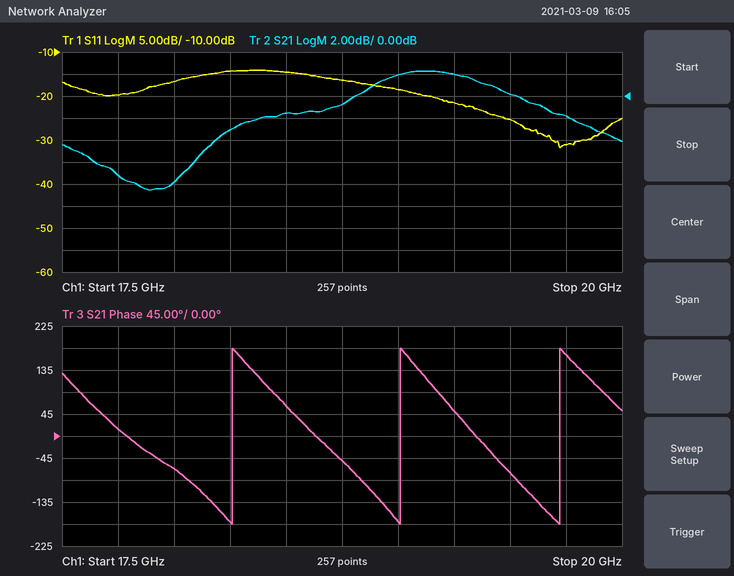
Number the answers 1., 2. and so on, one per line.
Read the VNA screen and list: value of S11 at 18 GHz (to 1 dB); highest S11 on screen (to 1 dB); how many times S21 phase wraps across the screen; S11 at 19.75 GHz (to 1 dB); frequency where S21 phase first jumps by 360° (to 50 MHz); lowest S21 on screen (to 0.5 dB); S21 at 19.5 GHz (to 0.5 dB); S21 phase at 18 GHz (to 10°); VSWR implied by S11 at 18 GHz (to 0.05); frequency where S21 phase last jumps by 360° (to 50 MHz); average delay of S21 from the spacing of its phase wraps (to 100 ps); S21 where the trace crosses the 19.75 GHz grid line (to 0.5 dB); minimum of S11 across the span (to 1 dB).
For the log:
1. -17 dB
2. -14 dB
3. 3
4. -31 dB
5. 18.25 GHz
6. -8.5 dB
7. 0.0 dB
8. -70°
9. 1.35
10. 19.70 GHz
11. 1.4 ns
12. -2.0 dB
13. -32 dB
